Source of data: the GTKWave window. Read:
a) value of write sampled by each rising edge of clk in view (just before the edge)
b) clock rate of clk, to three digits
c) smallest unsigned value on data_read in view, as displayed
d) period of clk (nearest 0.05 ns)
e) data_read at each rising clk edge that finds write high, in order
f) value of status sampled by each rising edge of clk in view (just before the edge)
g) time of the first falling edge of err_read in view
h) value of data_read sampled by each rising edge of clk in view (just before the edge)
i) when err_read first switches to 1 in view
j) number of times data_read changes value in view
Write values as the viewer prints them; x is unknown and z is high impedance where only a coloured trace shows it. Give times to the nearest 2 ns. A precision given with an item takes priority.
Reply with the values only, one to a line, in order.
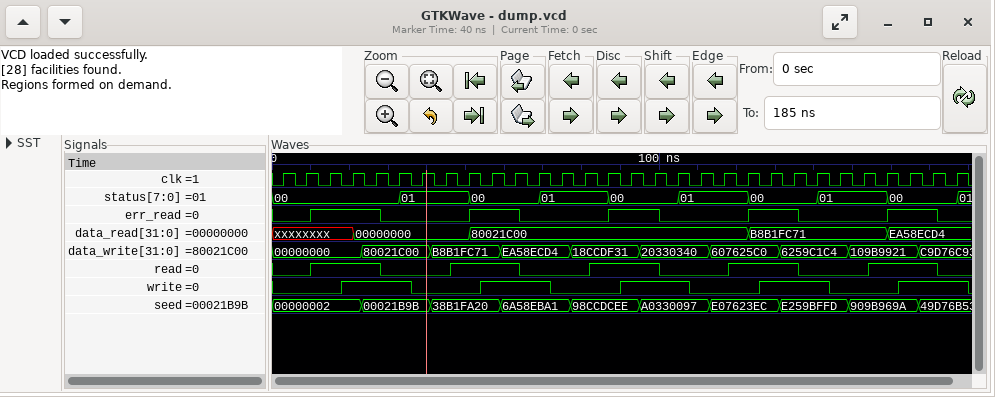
0 0 0 1 1 1 0 0 0 1 1 1 0 0 0 1 1 1 0 0 0 1 1 1 0 0 0 1 1 1
167 MHz
00000000
6 ns
xxxxxxxx, 00000000, 00000000, 80021C00, 80021C00, 80021C00, 80021C00, 80021C00, 80021C00, B8B1FC71, B8B1FC71, B8B1FC71, EA58ECD4, EA58ECD4, EA58ECD4
00, 00, 00, 00, 00, 00, 01, 01, 01, 00, 00, 00, 01, 01, 01, 00, 00, 00, 01, 01, 01, 00, 00, 00, 01, 01, 01, 00, 00, 00
28 ns
xxxxxxxx, xxxxxxxx, xxxxxxxx, xxxxxxxx, 00000000, 00000000, 00000000, 00000000, 00000000, 80021C00, 80021C00, 80021C00, 80021C00, 80021C00, 80021C00, 80021C00, 80021C00, 80021C00, 80021C00, 80021C00, 80021C00, B8B1FC71, B8B1FC71, B8B1FC71, B8B1FC71, B8B1FC71, B8B1FC71, EA58ECD4, EA58ECD4, EA58ECD4
10 ns
4
